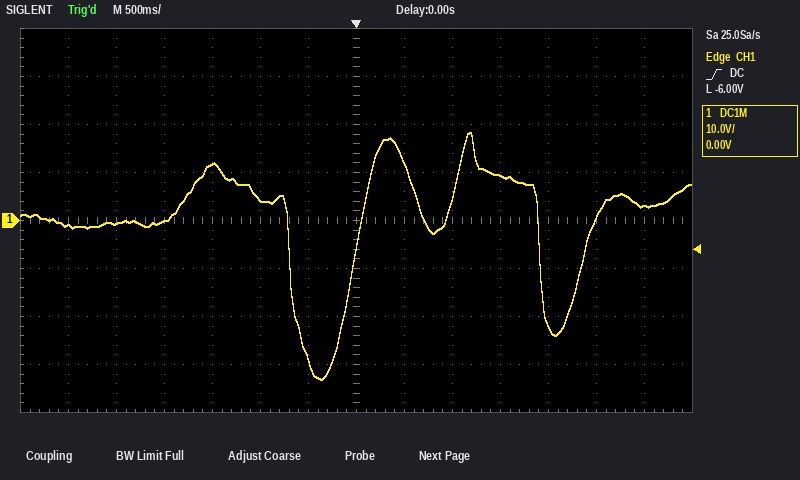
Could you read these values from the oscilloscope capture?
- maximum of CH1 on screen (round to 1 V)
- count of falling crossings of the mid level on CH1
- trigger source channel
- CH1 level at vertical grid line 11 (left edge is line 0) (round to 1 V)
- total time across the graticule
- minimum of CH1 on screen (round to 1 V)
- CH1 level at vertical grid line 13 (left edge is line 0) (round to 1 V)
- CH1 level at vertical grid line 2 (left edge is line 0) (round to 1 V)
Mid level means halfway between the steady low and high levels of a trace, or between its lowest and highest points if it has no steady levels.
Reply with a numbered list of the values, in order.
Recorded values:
1. 18 V
2. 2
3. CH1
4. -22 V
5. 7 s
6. -33 V
7. 3 V
8. -1 V
